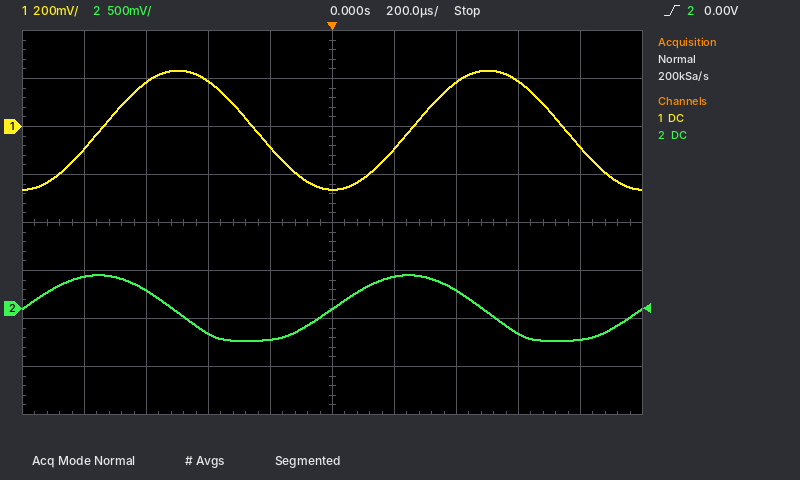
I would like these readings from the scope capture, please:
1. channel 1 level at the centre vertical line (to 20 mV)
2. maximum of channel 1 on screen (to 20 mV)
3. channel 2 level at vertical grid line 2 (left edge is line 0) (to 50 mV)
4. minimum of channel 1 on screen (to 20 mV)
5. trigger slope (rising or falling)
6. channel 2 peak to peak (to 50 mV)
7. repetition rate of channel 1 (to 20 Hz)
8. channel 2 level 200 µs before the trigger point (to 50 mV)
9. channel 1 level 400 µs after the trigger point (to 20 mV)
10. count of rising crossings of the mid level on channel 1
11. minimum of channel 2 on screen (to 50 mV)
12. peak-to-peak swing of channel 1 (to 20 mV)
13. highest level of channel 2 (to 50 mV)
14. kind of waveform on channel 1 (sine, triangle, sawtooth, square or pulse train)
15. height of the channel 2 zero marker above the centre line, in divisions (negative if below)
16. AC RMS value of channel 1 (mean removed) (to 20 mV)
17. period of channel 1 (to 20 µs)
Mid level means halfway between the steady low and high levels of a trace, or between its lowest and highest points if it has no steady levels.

-260 mV
240 mV
200 mV
-260 mV
rising
700 mV
1.00 kHz
-300 mV
180 mV
2
-350 mV
500 mV
350 mV
sine
-1.8 div
180 mV
1.00 ms
